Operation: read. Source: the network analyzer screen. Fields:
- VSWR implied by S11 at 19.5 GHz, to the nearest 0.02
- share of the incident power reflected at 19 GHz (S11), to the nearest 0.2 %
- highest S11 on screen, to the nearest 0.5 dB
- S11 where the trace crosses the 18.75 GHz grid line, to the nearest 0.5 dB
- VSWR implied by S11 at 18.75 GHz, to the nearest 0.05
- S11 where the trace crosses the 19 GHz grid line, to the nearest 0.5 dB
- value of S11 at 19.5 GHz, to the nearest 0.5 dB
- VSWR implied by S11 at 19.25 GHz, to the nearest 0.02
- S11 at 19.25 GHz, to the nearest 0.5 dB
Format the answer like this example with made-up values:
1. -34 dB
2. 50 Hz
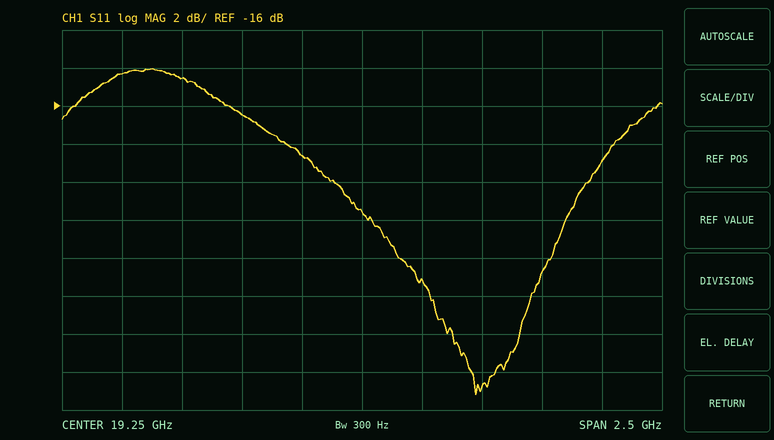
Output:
1. 1.12
2. 1.4 %
3. -14.0 dB
4. -16.5 dB
5. 1.35
6. -18.5 dB
7. -25.0 dB
8. 1.18
9. -21.5 dB
